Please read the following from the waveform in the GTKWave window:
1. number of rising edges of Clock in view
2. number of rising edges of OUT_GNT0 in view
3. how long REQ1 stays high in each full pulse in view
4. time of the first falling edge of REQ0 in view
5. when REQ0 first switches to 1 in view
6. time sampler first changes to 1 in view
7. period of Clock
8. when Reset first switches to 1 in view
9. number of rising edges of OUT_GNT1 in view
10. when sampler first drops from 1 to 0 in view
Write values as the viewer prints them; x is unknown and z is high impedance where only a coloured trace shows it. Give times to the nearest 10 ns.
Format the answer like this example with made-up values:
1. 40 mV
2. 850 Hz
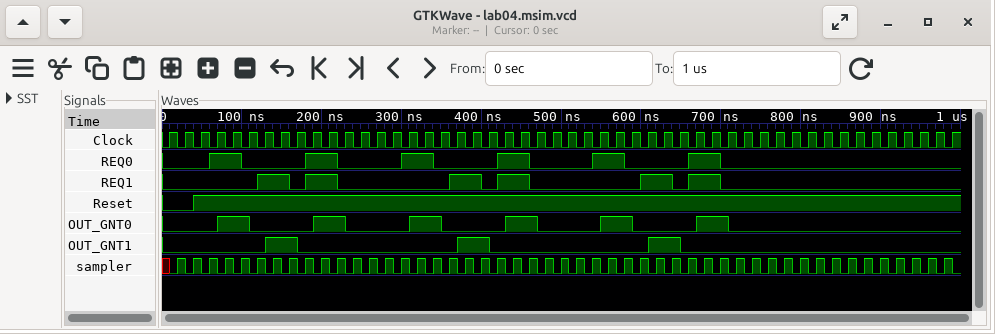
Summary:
1. 50
2. 6
3. 40 ns, 40 ns, 40 ns, 40 ns, 40 ns, 40 ns
4. 100 ns
5. 60 ns
6. 20 ns
7. 20 ns
8. 40 ns
9. 3
10. 30 ns
